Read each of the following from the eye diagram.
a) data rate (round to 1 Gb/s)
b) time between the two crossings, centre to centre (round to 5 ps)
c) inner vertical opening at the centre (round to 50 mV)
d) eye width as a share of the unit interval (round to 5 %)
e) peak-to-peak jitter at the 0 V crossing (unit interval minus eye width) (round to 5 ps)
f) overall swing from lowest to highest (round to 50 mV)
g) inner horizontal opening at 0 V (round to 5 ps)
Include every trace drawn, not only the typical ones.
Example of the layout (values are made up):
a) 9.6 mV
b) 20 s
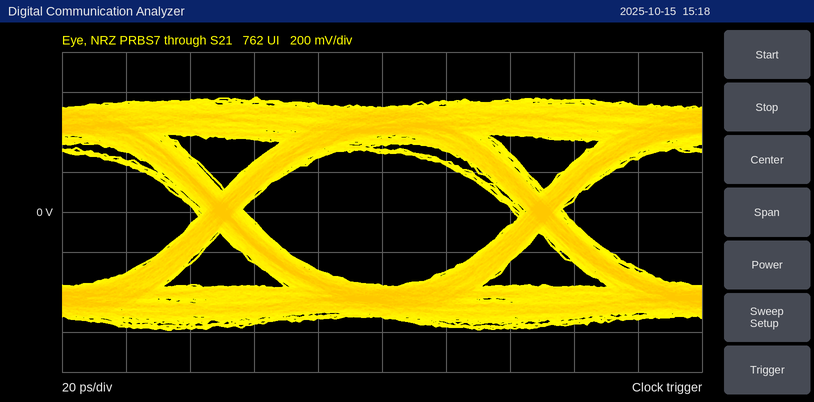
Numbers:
a) 10 Gb/s
b) 100 ps
c) 650 mV
d) 85 %
e) 15 ps
f) 1.15 V
g) 85 ps
